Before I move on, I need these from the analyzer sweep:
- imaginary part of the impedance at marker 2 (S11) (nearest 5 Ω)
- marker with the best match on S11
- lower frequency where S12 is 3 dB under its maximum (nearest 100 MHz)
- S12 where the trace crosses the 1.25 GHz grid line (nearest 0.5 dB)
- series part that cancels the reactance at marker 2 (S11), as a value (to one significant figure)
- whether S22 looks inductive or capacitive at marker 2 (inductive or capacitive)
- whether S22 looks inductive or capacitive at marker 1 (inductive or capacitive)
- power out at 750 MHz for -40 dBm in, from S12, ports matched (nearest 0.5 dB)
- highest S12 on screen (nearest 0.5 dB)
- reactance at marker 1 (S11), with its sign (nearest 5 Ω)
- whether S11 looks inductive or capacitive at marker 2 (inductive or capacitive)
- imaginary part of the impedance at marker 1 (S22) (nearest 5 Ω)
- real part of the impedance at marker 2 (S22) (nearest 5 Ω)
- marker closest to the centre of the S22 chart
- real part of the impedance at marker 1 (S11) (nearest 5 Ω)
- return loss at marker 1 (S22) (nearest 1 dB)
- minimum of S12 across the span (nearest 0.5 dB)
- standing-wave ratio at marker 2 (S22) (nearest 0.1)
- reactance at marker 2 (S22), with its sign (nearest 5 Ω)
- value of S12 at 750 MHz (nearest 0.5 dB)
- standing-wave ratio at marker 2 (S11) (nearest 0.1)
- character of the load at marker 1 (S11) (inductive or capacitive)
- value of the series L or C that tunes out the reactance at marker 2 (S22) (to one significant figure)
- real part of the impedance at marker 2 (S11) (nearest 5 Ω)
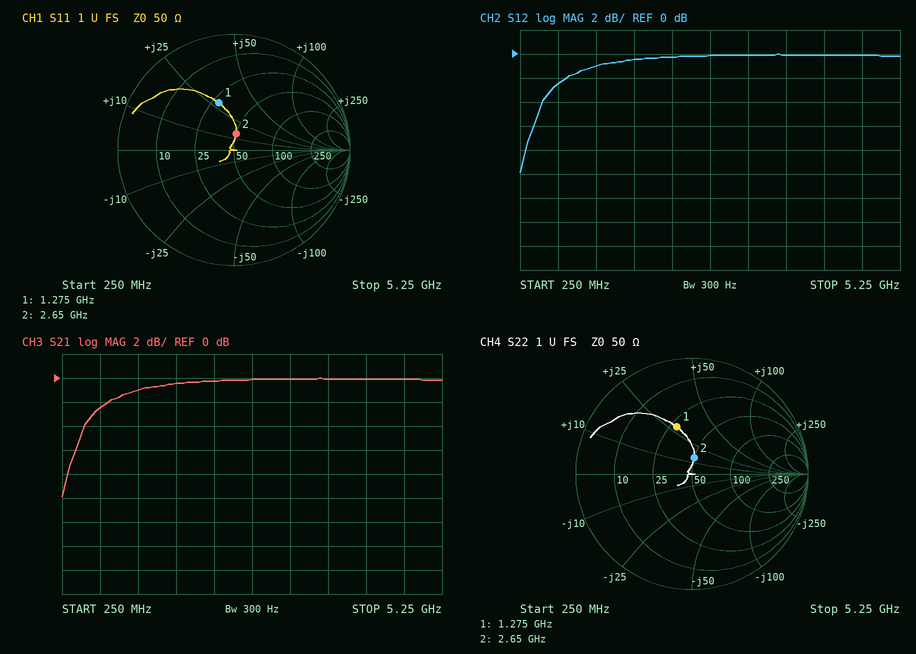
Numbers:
+15 Ω
marker 2
700 MHz
-1.0 dB
4 pF
inductive
inductive
-42.5 dBm
0.0 dB
+30 Ω
inductive
+30 Ω
50 Ω
marker 2
30 Ω
7 dB
-10.0 dB
1.3
+15 Ω
-2.5 dB
1.3
inductive
4 pF
50 Ω
